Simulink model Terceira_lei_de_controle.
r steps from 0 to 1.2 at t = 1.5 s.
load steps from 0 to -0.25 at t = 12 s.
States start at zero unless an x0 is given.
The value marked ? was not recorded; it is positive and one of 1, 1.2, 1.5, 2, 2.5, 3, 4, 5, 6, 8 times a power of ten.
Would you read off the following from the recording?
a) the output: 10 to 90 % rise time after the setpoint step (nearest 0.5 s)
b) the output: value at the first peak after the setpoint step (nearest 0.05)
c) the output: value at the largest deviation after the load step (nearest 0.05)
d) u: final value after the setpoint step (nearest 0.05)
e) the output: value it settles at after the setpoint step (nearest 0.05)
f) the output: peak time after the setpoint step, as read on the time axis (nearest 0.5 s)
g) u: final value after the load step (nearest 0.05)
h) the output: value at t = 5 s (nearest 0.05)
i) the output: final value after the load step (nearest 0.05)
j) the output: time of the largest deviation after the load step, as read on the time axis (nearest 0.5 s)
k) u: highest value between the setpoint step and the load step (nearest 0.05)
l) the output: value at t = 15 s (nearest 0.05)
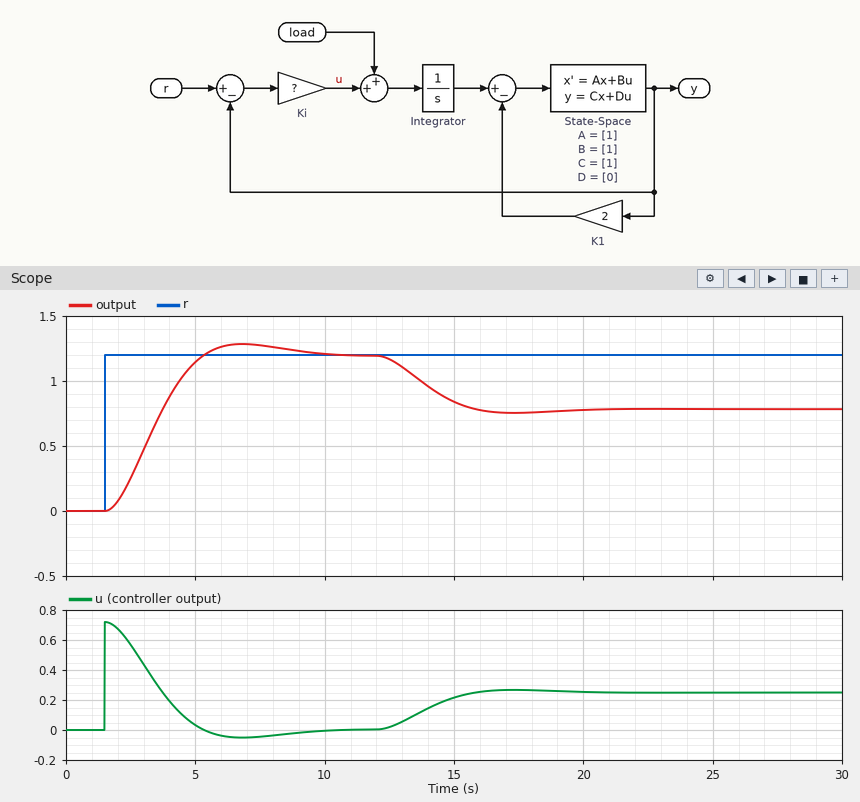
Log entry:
2.5 s
1.30
0.75
0.00
1.20
7.0 s
0.25
1.15
0.80
17.5 s
0.70
0.85
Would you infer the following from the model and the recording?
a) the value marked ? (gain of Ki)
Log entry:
0.6
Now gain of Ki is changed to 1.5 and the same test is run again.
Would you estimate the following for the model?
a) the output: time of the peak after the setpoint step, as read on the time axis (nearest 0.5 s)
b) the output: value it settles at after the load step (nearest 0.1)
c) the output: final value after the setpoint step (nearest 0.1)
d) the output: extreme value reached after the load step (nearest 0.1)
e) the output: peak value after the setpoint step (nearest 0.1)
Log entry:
4.5 s
1.0
1.2
1.0
1.5
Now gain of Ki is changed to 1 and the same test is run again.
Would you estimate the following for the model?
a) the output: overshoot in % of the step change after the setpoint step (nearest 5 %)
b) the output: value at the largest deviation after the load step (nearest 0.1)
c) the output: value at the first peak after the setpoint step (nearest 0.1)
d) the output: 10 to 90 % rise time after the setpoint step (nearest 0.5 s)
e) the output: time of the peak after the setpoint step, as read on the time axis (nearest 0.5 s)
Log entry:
15 %
0.9
1.4
1.5 s
5.0 s
